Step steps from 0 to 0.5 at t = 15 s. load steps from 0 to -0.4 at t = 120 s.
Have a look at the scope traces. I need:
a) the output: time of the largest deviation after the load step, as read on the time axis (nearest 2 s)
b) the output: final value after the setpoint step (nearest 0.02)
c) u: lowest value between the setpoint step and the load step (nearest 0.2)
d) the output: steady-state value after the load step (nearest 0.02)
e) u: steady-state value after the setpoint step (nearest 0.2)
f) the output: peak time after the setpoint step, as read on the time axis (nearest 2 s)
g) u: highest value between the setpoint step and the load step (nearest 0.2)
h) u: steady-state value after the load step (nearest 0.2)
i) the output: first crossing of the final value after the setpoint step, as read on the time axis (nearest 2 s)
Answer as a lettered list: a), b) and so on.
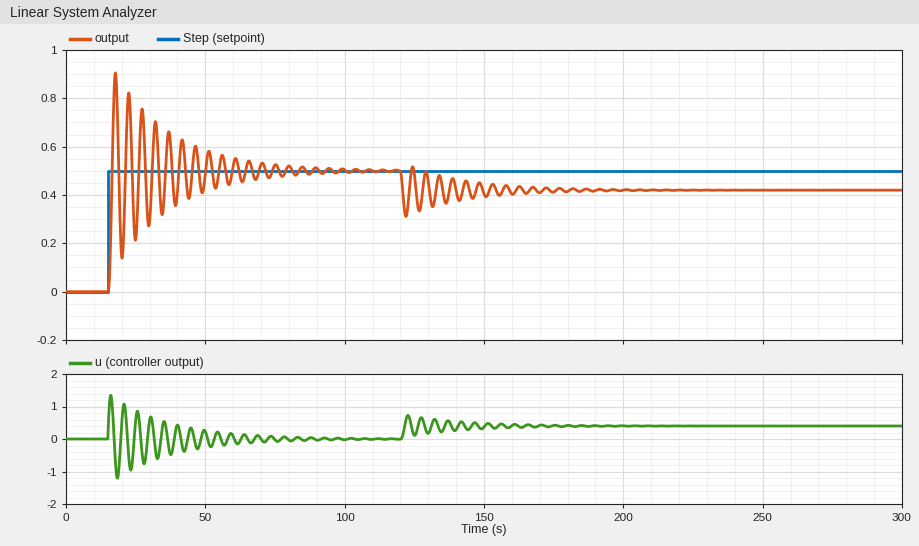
a) 122 s
b) 0.50
c) -1.2
d) 0.42
e) 0.0
f) 18 s
g) 1.4
h) 0.4
i) 16 s
